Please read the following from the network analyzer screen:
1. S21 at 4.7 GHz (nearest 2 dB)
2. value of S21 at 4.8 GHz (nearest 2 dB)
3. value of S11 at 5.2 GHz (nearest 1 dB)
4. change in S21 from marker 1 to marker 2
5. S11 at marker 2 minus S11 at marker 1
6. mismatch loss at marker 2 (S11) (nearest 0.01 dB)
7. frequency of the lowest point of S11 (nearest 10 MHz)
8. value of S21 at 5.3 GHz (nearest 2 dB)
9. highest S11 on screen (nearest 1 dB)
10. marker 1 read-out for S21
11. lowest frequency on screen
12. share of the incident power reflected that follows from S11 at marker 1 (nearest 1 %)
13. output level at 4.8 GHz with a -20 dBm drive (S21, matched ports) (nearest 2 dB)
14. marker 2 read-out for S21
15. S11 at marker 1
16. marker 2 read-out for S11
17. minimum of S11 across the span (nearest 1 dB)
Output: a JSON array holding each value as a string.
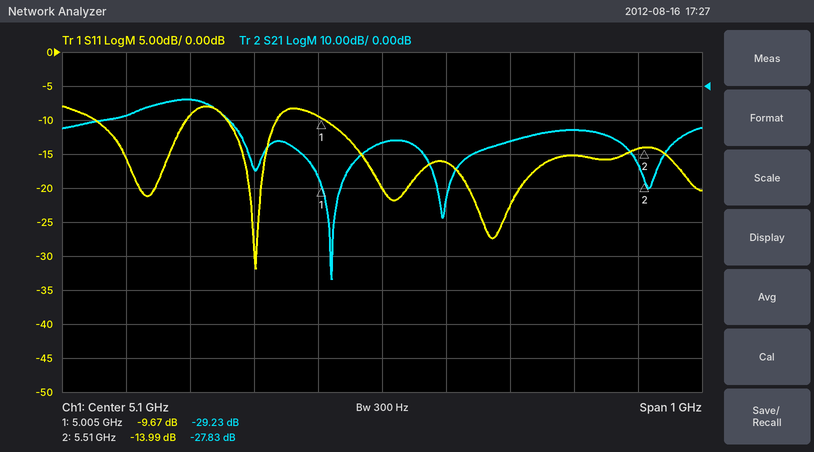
["-8 dB", "-4 dB", "-16 dB", "1.40 dB", "-4.32 dB", "0.18 dB", "4.90 GHz", "-16 dB", "-8 dB", "-29.23 dB", "4.6 GHz", "11 %", "-24 dBm", "-27.83 dB", "-9.67 dB", "-13.99 dB", "-32 dB"]
